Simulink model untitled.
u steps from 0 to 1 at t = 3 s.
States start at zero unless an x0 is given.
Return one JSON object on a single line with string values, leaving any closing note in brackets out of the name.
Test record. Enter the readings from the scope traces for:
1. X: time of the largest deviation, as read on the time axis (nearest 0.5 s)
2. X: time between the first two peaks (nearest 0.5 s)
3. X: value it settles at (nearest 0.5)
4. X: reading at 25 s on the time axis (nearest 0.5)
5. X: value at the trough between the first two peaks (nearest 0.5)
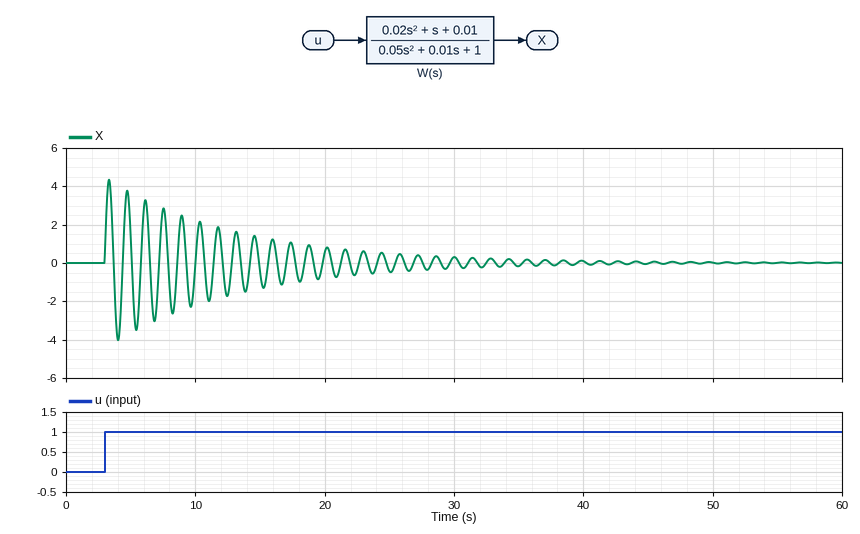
{"X: time of the largest deviation, as read on the time axis": "3.5 s", "X: time between the first two peaks": "1.5 s", "X: value it settles at": "0.0", "X: reading at 25 s on the time axis": "-0.5", "X: value at the trough between the first two peaks": "-4.0"}
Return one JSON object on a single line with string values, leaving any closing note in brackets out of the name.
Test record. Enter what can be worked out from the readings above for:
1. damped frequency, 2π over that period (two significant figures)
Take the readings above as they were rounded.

{"damped frequency, 2π over that period": "4.2 rad/s"}
